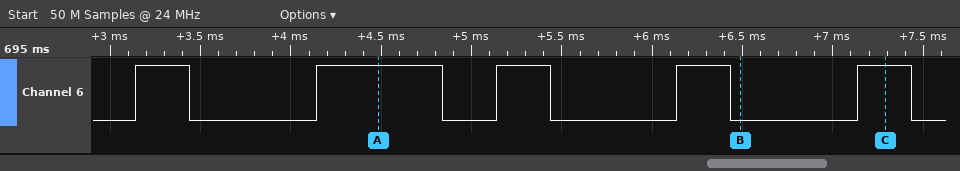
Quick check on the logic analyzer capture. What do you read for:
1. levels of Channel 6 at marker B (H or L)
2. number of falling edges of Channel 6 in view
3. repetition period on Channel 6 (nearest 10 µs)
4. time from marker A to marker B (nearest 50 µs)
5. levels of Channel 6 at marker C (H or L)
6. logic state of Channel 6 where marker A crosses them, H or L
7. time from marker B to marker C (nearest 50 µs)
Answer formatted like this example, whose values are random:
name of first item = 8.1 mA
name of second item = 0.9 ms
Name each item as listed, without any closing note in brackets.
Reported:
levels of Channel 6 at marker B = Channel 6=L
number of falling edges of Channel 6 in view = 5
repetition period on Channel 6 = 1000 µs
time from marker A to marker B = 2000 µs
levels of Channel 6 at marker C = Channel 6=H
logic state of Channel 6 where marker A crosses them, H or L = Channel 6=H
time from marker B to marker C = 800 µs
